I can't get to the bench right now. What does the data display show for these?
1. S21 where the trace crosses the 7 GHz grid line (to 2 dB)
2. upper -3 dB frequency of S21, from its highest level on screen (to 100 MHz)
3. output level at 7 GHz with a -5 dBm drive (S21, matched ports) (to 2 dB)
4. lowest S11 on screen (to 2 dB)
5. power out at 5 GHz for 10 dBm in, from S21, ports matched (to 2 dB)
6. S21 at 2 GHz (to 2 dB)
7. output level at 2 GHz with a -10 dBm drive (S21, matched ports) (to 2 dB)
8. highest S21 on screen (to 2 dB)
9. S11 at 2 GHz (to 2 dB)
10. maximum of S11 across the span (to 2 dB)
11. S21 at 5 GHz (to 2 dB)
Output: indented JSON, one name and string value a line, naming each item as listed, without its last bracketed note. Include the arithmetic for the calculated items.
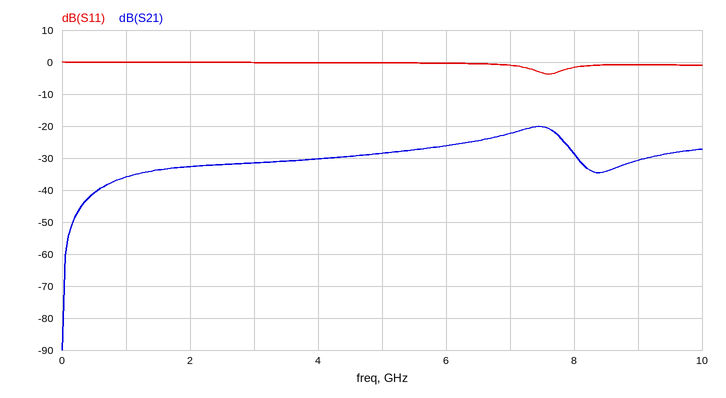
{
  "S21 where the trace crosses the 7 GHz grid line": "-22 dB",
  "upper -3 dB frequency of S21, from its highest level on screen": "7.8 GHz",
  "output level at 7 GHz with a -5 dBm drive (S21, matched ports)": "-5 dBm + (-22 dB) = -28 dBm",
  "lowest S11 on screen": "-4 dB",
  "power out at 5 GHz for 10 dBm in, from S21, ports matched": "10 dBm + (-28 dB) = -18 dBm",
  "S21 at 2 GHz": "-32 dB",
  "output level at 2 GHz with a -10 dBm drive (S21, matched ports)": "-10 dBm + (-32 dB) = -42 dBm",
  "highest S21 on screen": "-20 dB",
  "S11 at 2 GHz": "0 dB",
  "maximum of S11 across the span": "0 dB",
  "S21 at 5 GHz": "-28 dB"
}
